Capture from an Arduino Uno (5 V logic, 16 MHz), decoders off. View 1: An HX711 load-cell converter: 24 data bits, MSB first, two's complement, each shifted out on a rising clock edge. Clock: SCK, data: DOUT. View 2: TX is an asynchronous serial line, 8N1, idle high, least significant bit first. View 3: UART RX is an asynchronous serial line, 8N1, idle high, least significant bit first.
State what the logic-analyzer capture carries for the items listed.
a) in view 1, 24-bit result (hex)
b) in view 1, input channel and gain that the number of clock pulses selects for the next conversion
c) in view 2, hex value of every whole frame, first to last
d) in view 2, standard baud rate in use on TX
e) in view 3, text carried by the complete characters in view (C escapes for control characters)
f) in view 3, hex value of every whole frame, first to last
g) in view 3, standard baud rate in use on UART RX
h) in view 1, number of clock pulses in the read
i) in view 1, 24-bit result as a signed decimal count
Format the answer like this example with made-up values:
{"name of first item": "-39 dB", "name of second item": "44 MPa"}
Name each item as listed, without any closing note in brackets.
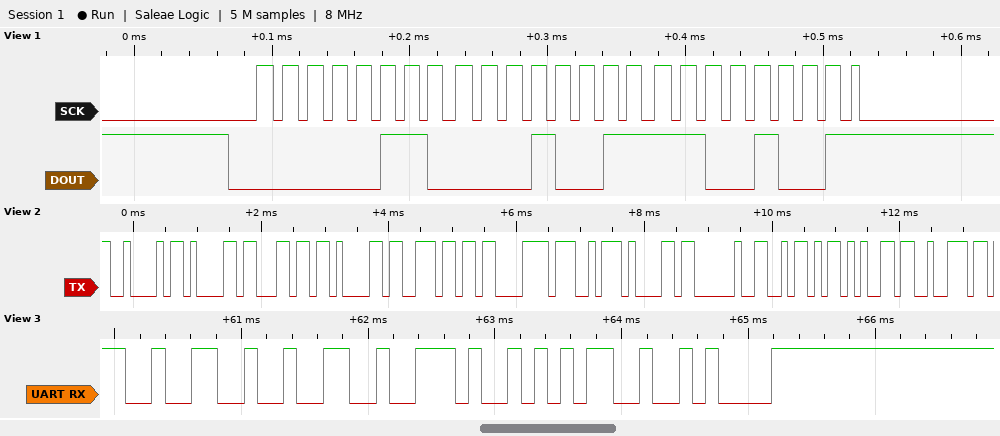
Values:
{"in view 1, 24-bit result": "0x0613C9", "in view 1, input channel and gain that the number of clock pulses selects for the next conversion": "channel A, gain 128", "in view 2, hex value of every whole frame, first to last": "42 61 6C 61 6E C3 A7 61 20 5A 65 72", "in view 2, standard baud rate in use on TX": "9600 baud", "in view 3, text carried by the complete characters in view": "\"22.5\\n\"", "in view 3, hex value of every whole frame, first to last": "32 32 2E 35 0A", "in view 3, standard baud rate in use on UART RX": "9600 baud", "in view 1, number of clock pulses in the read": "25", "in view 1, 24-bit result as a signed decimal count": "398281"}
